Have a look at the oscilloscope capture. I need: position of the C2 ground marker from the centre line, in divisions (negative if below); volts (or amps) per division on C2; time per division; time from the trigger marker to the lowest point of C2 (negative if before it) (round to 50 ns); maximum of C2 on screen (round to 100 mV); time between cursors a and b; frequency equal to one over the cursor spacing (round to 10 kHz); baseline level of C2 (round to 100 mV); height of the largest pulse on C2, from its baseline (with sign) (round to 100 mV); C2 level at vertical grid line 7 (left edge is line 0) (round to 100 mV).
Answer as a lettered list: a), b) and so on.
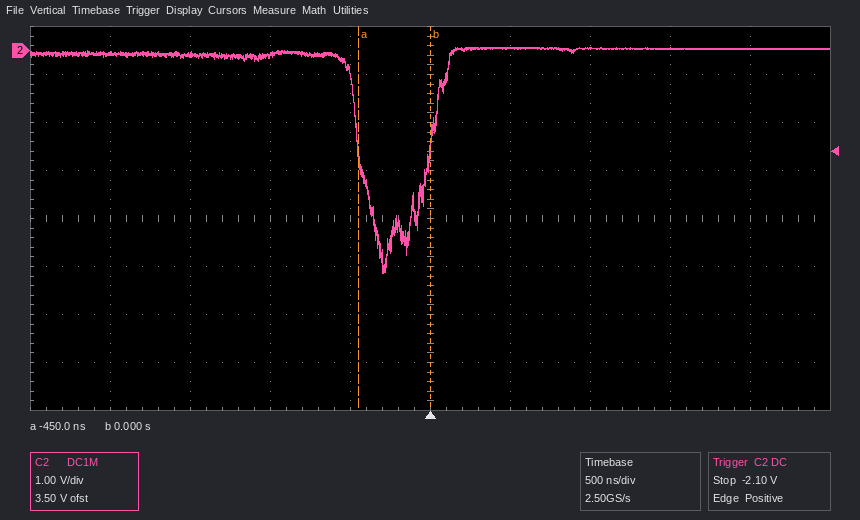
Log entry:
a) +3.5 div
b) 1 V
c) 500 ns
d) -300 ns
e) 100 mV
f) 450 ns
g) 2.22 MHz
h) 0.0 V
i) -4.7 V
j) 0.0 V
